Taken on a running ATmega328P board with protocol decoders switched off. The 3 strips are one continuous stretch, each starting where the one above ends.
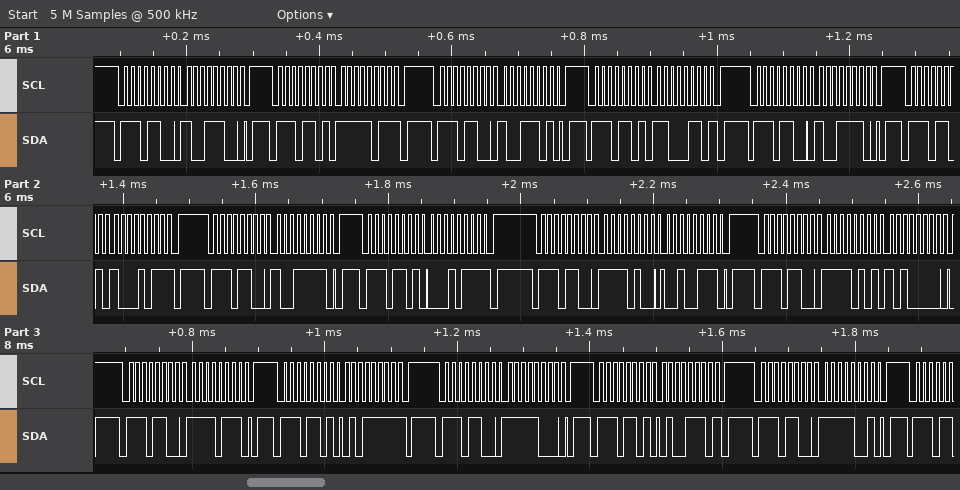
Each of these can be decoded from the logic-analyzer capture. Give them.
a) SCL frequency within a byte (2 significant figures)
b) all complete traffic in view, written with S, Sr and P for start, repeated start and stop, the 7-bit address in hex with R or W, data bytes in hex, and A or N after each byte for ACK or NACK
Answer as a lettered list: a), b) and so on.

a) 100 kHz
b) S 76W A 9C A P S 76R A FB N P S 76W A 9D A P S 76R A C6 N P S 76W A 9E A P S 76R A 8B N P S 76W A 9F A P S 76R A 17 N P S 76W A F4 A 27 A P S 76W A F5 A A0 A P S 76W A F7 A P S 76R A 5F N P S 76W A F8 A P S 76R A 4E N P S 76W A F9 A P
